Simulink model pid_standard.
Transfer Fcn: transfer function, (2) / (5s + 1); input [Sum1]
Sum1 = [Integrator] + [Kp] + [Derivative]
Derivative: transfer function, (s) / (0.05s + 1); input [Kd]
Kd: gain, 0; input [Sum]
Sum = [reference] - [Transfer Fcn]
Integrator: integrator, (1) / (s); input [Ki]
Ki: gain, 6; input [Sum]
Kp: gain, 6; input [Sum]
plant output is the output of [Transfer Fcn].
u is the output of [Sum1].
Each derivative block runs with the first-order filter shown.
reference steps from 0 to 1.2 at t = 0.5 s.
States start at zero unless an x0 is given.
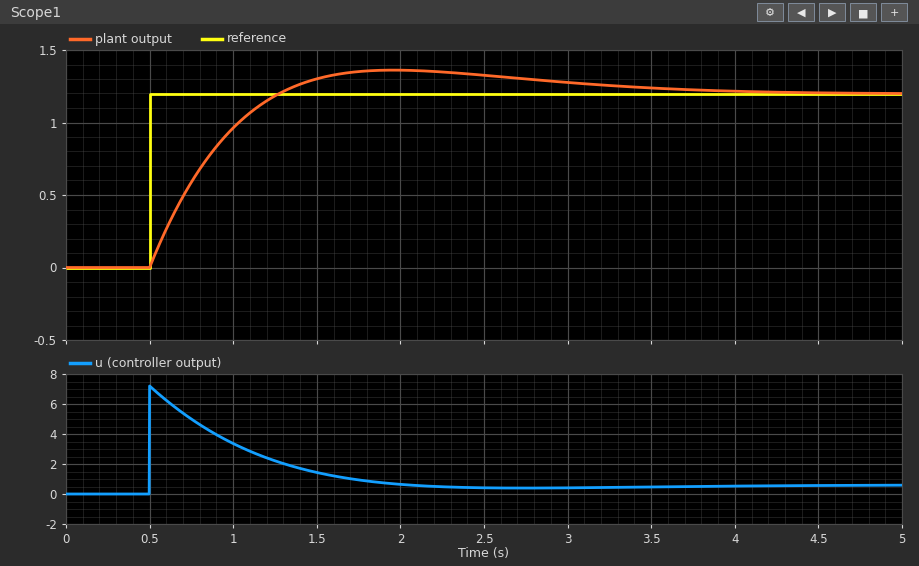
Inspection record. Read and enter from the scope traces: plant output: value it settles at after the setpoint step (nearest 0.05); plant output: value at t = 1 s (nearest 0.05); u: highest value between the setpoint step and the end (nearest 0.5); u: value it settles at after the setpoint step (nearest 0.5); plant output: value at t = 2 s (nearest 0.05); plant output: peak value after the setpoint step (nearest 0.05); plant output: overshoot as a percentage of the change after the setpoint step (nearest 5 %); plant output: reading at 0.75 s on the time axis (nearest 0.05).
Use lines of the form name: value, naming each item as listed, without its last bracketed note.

plant output: value it settles at after the setpoint step: 1.20
plant output: value at t = 1 s: 0.95
u: highest value between the setpoint step and the end: 7.0
u: value it settles at after the setpoint step: 0.5
plant output: value at t = 2 s: 1.35
plant output: peak value after the setpoint step: 1.35
plant output: overshoot as a percentage of the change after the setpoint step: 15 %
plant output: reading at 0.75 s on the time axis: 0.60
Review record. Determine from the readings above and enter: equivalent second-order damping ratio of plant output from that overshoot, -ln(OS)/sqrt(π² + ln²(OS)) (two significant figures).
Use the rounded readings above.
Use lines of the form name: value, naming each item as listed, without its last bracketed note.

equivalent second-order damping ratio of plant output from that overshoot, -ln(OS)/sqrt(π² + ln²(OS)): 0.52
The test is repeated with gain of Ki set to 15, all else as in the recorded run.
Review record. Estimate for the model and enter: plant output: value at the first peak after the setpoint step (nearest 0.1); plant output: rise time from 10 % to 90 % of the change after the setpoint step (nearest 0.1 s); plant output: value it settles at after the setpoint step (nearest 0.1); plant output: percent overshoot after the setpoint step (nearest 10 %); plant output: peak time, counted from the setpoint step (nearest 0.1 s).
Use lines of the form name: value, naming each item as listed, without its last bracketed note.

plant output: value at the first peak after the setpoint step: 1.5
plant output: rise time from 10 % to 90 % of the change after the setpoint step: 0.4 s
plant output: value it settles at after the setpoint step: 1.2
plant output: percent overshoot after the setpoint step: 30 %
plant output: peak time, counted from the setpoint step: 1.0 s
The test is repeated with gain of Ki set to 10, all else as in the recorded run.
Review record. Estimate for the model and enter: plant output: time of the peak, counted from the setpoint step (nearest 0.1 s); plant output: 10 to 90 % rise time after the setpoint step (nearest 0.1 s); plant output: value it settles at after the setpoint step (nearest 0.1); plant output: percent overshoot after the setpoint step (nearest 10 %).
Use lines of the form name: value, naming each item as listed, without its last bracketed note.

plant output: time of the peak, counted from the setpoint step: 1.2 s
plant output: 10 to 90 % rise time after the setpoint step: 0.5 s
plant output: value it settles at after the setpoint step: 1.2
plant output: percent overshoot after the setpoint step: 20 %
